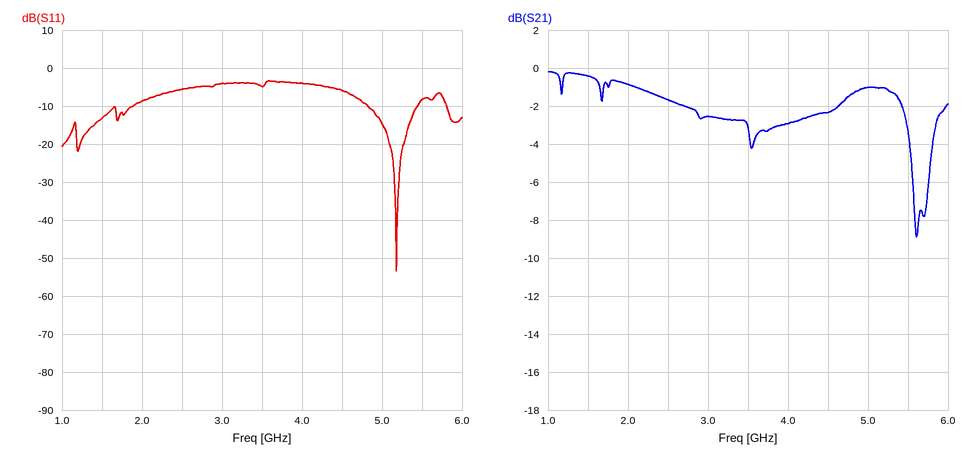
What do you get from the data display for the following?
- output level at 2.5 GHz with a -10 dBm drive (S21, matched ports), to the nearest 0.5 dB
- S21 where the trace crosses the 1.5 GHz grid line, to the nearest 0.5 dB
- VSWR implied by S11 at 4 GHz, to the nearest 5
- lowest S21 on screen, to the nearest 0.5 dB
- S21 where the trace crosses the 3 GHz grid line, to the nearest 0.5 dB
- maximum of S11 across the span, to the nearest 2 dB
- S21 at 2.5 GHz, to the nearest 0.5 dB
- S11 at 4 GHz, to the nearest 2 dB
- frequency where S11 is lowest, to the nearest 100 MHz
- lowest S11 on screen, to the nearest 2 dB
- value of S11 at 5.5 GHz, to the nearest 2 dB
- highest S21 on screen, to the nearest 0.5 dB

-11.5 dBm
-0.5 dB
5
-9.0 dB
-2.5 dB
-4 dB
-1.5 dB
-4 dB
5.2 GHz
-54 dB
-8 dB
0.0 dB
